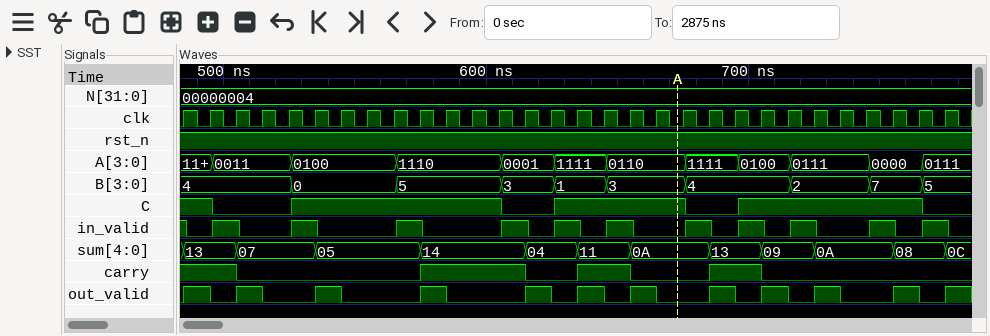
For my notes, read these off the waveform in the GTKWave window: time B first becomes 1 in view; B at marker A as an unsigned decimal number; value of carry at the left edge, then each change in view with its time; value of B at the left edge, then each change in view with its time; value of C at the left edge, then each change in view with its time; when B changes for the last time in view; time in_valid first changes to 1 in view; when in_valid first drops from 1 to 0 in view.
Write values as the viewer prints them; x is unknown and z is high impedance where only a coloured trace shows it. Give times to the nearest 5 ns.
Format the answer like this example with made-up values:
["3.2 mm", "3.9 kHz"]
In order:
["625 ns", "3", "1, 0 at 505 ns, 1 at 575 ns, 0 at 615 ns, 1 at 635 ns, 0 at 655 ns, 1 at 685 ns, 0 at 705 ns", "4, 0 at 525 ns, 5 at 565 ns, 3 at 605 ns, 1 at 625 ns, 3 at 645 ns, 4 at 675 ns, 2 at 715 ns, 7 at 745 ns, 5 at 765 ns", "1, 0 at 495 ns, 1 at 525 ns, 0 at 605 ns, 1 at 625 ns, 0 at 675 ns, 1 at 695 ns, 0 at 765 ns", "765 ns", "495 ns", "485 ns"]
